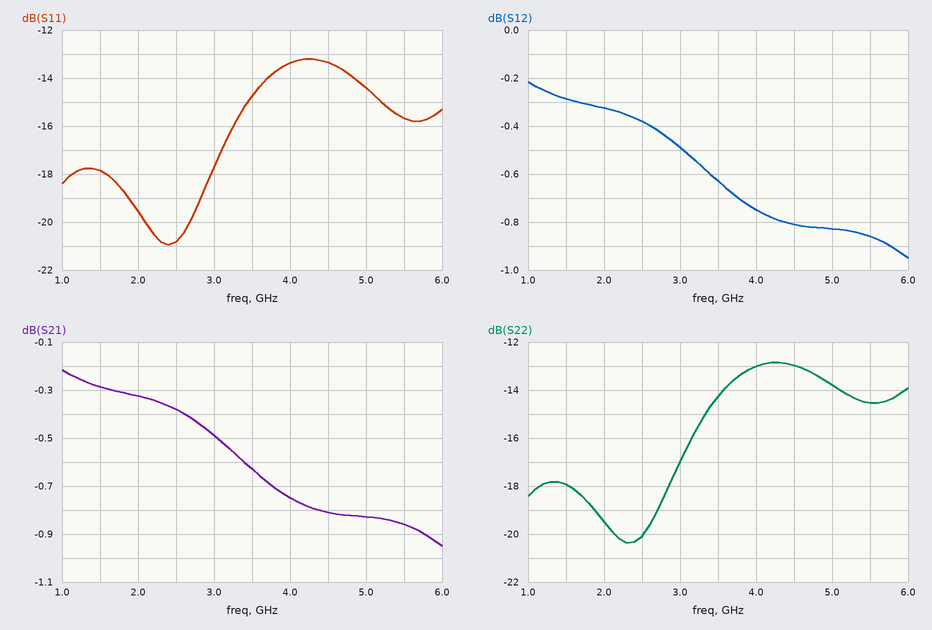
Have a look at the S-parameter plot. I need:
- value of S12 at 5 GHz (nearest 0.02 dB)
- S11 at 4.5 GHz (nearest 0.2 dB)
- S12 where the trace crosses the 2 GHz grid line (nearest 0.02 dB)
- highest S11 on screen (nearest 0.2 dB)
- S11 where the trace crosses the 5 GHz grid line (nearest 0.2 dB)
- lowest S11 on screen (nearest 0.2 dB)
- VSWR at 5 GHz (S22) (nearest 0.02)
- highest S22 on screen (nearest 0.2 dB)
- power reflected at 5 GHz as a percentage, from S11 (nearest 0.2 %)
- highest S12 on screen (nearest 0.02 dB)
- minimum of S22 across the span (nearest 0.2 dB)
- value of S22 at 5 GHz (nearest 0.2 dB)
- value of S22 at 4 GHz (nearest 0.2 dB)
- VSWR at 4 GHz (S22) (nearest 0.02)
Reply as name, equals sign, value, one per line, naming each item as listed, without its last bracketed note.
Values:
value of S12 at 5 GHz = -0.82 dB
S11 at 4.5 GHz = -13.4 dB
S12 where the trace crosses the 2 GHz grid line = -0.32 dB
highest S11 on screen = -13.2 dB
S11 where the trace crosses the 5 GHz grid line = -14.4 dB
lowest S11 on screen = -21.0 dB
VSWR at 5 GHz (S22) = 1.52
highest S22 on screen = -12.8 dB
power reflected at 5 GHz as a percentage, from S11 = 3.6 %
highest S12 on screen = -0.22 dB
minimum of S22 across the span = -20.4 dB
value of S22 at 5 GHz = -13.8 dB
value of S22 at 4 GHz = -13.0 dB
VSWR at 4 GHz (S22) = 1.58
